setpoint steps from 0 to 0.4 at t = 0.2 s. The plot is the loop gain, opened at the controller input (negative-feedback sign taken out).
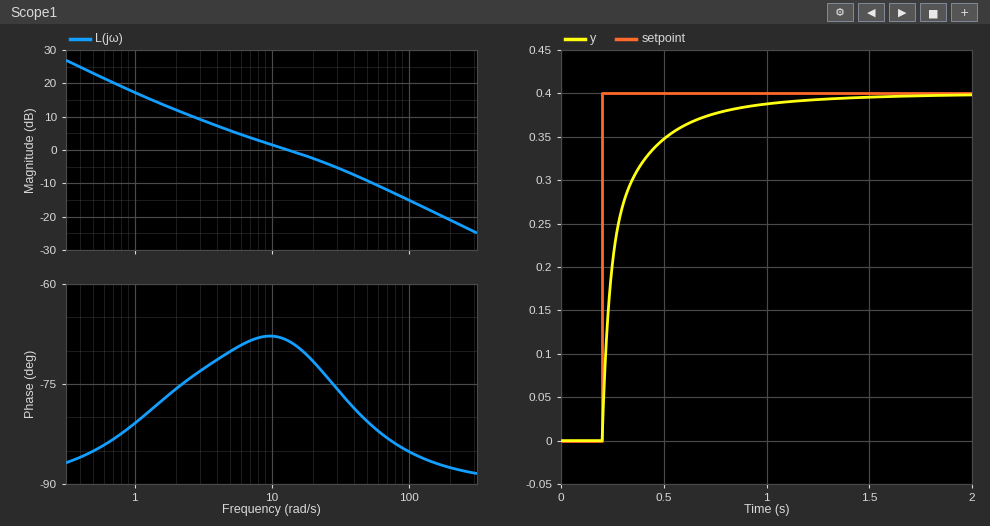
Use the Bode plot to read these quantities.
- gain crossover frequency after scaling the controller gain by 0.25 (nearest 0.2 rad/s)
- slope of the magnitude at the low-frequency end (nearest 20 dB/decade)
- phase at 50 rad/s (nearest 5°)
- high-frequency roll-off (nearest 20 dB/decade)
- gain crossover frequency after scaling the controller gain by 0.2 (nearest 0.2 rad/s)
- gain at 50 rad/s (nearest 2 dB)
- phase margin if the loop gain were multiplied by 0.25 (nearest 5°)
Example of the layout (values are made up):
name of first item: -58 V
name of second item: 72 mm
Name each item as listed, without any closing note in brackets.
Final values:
gain crossover frequency after scaling the controller gain by 0.25: 2.0 rad/s
slope of the magnitude at the low-frequency end: -20 dB/decade
phase at 50 rad/s: -80°
high-frequency roll-off: -20 dB/decade
gain crossover frequency after scaling the controller gain by 0.2: 1.6 rad/s
gain at 50 rad/s: -10 dB
phase margin if the loop gain were multiplied by 0.25: 105°
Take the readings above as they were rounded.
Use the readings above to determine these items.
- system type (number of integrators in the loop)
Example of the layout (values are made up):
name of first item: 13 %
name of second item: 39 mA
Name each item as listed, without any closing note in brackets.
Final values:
system type: 1
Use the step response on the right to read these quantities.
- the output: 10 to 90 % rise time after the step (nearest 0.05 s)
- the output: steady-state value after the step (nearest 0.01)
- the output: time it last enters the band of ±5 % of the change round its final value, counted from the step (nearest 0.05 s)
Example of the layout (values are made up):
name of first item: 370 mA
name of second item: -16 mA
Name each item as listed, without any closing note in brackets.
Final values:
the output: 10 to 90 % rise time after the step: 0.35 s
the output: steady-state value after the step: 0.40
the output: time it last enters the band of ±5 % of the change round its final value, counted from the step: 0.60 s
